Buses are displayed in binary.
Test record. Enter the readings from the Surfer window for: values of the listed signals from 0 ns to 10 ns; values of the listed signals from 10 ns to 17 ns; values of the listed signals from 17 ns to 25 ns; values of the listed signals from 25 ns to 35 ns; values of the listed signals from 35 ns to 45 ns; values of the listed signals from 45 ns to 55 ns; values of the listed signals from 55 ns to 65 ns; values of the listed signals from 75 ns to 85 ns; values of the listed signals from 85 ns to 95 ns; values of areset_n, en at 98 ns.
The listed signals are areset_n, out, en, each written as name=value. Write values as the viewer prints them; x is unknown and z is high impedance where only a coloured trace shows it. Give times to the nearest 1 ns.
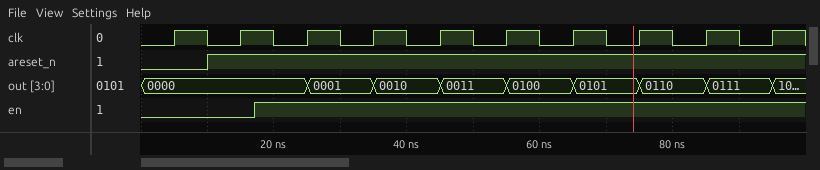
areset_n=0, out=0000, en=0
areset_n=1, out=0000, en=0
areset_n=1, out=0000, en=1
areset_n=1, out=0001, en=1
areset_n=1, out=0010, en=1
areset_n=1, out=0011, en=1
areset_n=1, out=0100, en=1
areset_n=1, out=0110, en=1
areset_n=1, out=0111, en=1
areset_n=1, en=1
